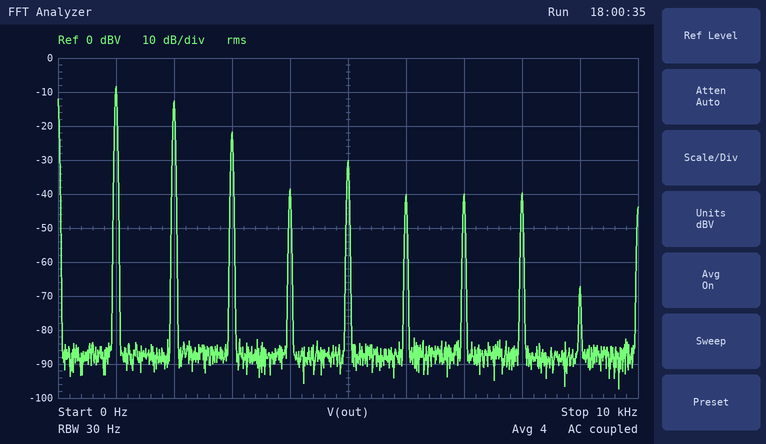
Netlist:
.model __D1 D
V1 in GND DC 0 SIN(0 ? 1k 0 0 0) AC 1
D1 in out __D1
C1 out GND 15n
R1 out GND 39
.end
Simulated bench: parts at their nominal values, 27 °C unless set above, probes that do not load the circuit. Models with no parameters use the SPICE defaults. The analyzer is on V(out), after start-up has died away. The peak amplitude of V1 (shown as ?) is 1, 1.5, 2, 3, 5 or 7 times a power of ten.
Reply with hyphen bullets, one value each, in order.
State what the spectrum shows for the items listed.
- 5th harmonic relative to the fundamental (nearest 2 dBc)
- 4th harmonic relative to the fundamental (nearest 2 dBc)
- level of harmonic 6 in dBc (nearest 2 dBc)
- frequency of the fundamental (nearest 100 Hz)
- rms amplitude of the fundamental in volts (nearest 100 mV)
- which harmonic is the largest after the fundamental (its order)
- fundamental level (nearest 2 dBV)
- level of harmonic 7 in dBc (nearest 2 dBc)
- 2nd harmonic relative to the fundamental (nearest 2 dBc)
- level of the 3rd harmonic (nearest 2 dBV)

- -22 dBc
- -30 dBc
- -32 dBc
- 1.0 kHz
- 400 mV
- 2
- -8 dBV
- -32 dBc
- -4 dBc
- -22 dBV
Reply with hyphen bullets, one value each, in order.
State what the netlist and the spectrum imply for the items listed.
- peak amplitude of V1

- 2 V
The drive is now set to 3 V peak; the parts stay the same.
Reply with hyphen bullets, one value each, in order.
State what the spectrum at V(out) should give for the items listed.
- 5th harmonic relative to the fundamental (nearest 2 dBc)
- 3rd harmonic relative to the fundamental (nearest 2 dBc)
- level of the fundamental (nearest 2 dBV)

- -24 dBc
- -18 dBc
- -2 dBV
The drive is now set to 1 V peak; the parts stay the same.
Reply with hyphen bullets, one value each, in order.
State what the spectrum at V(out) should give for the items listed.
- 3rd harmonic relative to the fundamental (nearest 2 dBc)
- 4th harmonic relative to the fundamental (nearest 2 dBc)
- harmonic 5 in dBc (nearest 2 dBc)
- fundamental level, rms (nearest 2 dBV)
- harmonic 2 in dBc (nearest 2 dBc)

- -6 dBc
- -12 dBc
- -26 dBc
- -24 dBV
- -2 dBc
